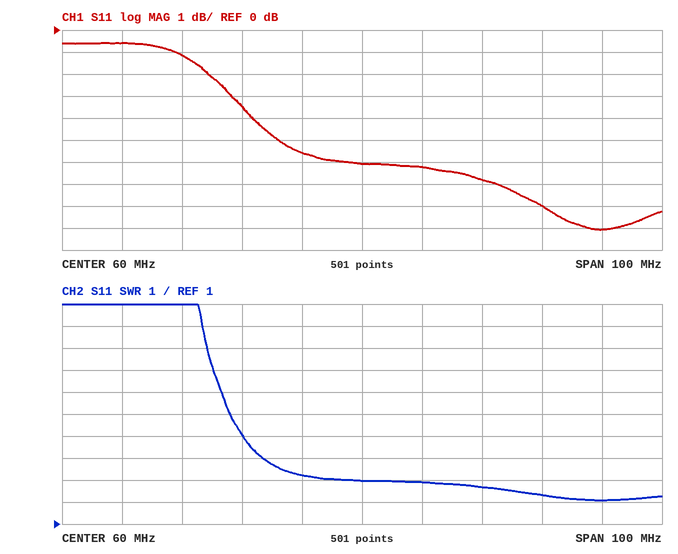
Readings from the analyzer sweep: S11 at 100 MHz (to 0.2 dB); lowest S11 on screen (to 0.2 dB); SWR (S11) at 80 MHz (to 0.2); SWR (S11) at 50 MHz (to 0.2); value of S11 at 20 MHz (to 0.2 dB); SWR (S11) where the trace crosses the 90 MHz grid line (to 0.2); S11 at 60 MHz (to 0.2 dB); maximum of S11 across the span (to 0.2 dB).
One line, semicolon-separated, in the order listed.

-9.0 dB; -9.0 dB; 2.6; 3.2; -0.6 dB; 2.4; -6.0 dB; -0.6 dB
